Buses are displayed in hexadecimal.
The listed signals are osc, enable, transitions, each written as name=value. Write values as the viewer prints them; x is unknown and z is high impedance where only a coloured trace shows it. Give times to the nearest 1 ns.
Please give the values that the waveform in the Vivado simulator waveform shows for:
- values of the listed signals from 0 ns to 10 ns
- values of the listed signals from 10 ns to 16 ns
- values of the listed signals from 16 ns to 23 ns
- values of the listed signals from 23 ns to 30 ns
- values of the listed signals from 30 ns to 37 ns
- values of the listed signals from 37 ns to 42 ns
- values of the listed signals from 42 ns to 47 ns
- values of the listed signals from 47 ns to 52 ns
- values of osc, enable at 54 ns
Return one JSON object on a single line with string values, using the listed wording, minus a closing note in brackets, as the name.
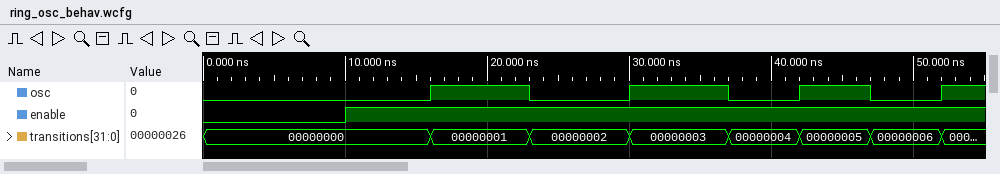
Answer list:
{"values of the listed signals from 0 ns to 10 ns": "osc=0, enable=0, transitions=00000000", "values of the listed signals from 10 ns to 16 ns": "osc=0, enable=1, transitions=00000000", "values of the listed signals from 16 ns to 23 ns": "osc=1, enable=1, transitions=00000001", "values of the listed signals from 23 ns to 30 ns": "osc=0, enable=1, transitions=00000002", "values of the listed signals from 30 ns to 37 ns": "osc=1, enable=1, transitions=00000003", "values of the listed signals from 37 ns to 42 ns": "osc=0, enable=1, transitions=00000004", "values of the listed signals from 42 ns to 47 ns": "osc=1, enable=1, transitions=00000005", "values of the listed signals from 47 ns to 52 ns": "osc=0, enable=1, transitions=00000006", "values of osc, enable at 54 ns": "osc=1, enable=1"}
